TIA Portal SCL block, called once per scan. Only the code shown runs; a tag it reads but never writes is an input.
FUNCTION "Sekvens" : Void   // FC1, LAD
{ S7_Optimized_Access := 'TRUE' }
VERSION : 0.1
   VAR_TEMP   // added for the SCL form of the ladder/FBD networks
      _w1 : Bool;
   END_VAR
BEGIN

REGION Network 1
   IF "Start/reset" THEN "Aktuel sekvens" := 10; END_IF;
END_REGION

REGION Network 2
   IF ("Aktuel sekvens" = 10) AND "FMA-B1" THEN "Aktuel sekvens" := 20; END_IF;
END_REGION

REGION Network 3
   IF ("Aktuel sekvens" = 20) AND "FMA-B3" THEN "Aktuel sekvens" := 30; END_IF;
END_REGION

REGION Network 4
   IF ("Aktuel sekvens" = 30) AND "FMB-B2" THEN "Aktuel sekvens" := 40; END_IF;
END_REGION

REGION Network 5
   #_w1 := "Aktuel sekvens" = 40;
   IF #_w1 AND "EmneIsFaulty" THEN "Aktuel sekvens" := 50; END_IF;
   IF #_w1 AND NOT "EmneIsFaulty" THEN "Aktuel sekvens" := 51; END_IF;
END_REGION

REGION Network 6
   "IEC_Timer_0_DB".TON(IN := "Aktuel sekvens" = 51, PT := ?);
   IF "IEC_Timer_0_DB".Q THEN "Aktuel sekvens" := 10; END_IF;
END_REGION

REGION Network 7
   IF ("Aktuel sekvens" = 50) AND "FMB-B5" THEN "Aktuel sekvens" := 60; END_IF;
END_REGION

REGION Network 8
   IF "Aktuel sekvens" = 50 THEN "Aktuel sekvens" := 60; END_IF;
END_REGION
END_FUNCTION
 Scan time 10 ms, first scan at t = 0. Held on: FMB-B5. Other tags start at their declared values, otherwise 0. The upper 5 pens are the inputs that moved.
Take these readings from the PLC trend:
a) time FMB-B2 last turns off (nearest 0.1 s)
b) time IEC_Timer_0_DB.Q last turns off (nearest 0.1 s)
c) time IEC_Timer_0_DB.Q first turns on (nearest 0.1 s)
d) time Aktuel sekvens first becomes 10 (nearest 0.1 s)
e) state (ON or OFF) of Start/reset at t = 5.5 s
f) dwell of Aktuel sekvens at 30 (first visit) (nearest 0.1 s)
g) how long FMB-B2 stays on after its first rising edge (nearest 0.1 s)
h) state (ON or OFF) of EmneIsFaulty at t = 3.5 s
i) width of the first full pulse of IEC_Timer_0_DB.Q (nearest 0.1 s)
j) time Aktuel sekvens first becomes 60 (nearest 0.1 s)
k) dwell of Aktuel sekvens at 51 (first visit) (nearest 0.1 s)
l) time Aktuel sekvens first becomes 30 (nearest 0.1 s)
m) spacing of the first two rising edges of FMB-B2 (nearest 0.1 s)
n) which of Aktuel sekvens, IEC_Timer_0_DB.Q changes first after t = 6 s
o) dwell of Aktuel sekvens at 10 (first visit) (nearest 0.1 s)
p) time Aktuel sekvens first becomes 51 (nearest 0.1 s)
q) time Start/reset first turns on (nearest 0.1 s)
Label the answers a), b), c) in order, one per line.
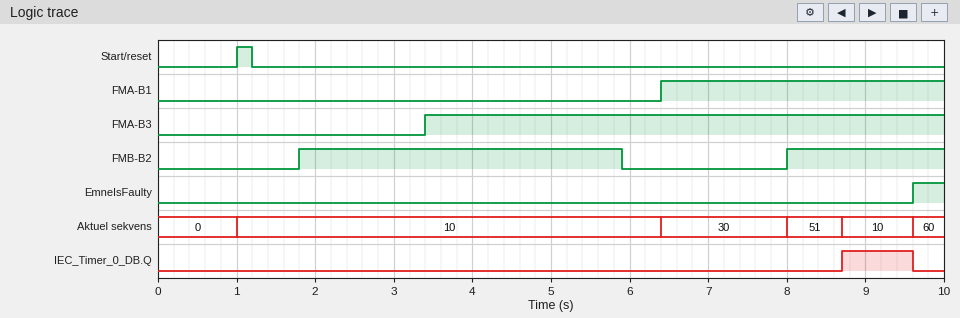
a) 5.9 s
b) 9.6 s
c) 8.7 s
d) 1.0 s
e) OFF
f) 1.6 s
g) 4.1 s
h) OFF
i) 0.9 s
j) 9.6 s
k) 0.7 s
l) 6.4 s
m) 6.2 s
n) Aktuel sekvens
o) 5.4 s
p) 8.0 s
q) 1.0 s
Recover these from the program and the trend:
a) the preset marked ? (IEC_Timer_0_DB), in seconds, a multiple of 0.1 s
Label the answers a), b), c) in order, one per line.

a) 0.7 s
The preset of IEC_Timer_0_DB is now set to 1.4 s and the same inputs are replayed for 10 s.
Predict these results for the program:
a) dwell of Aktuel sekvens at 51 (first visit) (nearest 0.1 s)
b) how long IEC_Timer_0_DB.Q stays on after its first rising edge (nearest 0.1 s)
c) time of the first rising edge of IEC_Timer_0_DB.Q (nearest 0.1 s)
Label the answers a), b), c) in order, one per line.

a) 1.4 s
b) 0.2 s
c) 9.4 s
